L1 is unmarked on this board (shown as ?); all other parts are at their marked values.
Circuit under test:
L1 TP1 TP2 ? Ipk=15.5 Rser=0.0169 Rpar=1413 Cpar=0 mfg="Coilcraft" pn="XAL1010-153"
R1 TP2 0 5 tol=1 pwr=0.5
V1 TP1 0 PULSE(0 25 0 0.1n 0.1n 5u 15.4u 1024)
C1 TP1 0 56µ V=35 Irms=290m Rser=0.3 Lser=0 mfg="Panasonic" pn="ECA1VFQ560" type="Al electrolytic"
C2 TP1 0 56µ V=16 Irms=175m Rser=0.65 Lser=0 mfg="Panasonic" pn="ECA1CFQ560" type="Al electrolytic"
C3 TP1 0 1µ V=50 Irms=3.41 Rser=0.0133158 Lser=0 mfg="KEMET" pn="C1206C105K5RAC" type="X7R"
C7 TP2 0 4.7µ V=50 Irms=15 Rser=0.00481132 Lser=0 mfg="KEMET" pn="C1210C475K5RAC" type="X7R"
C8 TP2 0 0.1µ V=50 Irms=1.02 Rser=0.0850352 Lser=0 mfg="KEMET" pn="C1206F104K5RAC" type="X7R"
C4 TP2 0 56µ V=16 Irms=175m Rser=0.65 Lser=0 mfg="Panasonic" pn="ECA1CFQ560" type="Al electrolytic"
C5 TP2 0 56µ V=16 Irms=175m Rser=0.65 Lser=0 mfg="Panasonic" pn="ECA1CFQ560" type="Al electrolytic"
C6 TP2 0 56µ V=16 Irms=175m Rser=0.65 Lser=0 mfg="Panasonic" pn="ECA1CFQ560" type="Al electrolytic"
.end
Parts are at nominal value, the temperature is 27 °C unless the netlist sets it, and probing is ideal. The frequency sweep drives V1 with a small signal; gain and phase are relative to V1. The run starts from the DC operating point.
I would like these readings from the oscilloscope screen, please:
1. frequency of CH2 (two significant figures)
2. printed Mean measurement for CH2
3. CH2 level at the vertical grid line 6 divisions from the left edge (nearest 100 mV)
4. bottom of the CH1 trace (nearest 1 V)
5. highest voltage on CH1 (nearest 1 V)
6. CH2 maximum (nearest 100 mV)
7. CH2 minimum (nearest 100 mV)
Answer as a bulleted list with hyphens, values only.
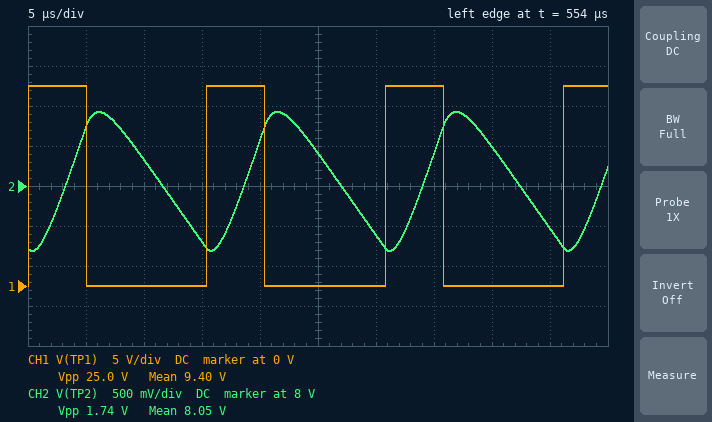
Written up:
- 65 kHz
- 8.05 V
- 7.4 V
- 0 V
- 25 V
- 8.9 V
- 7.2 V
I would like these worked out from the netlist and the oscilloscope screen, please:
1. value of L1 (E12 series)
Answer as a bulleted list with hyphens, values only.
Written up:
- 8.2 µH
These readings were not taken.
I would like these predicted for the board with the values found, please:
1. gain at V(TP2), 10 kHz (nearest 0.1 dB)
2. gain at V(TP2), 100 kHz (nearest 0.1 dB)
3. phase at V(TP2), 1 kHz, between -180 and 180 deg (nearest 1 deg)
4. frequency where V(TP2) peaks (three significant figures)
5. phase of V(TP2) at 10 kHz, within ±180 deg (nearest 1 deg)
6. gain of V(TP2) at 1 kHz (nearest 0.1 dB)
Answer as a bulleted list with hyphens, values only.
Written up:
- -6.6 dB
- -29.4 dB
- -2 deg
- 3.48 kHz
- -89 deg
- 0.4 dB
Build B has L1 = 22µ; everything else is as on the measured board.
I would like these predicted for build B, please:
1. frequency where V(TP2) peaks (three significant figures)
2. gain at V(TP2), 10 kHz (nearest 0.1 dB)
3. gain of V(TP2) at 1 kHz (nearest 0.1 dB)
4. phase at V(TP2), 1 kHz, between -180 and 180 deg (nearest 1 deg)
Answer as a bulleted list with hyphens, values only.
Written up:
- 2.31 kHz
- -15.4 dB
- 1.2 dB
- -5 deg
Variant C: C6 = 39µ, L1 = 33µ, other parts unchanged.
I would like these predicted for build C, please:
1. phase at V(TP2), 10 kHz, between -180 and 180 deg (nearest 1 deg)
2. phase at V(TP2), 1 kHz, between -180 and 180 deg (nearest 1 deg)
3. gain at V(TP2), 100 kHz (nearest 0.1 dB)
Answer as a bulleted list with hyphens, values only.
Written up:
- -112 deg
- -7 deg
- -41.6 dB
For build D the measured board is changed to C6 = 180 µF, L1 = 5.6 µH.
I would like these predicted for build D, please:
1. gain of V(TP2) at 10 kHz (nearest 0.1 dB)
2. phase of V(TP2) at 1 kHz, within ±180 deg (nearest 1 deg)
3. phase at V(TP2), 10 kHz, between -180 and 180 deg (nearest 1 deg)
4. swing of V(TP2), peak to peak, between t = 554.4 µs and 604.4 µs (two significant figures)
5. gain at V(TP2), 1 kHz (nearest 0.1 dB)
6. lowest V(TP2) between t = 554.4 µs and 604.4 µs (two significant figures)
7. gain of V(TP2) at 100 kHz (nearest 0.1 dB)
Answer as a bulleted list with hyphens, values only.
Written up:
- -4.2 dB
- -3 deg
- -72 deg
- 2.6 V
- 0.3 dB
- 6.8 V
- -26.0 dB
